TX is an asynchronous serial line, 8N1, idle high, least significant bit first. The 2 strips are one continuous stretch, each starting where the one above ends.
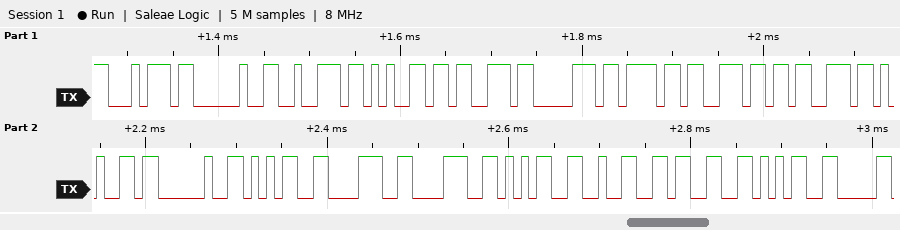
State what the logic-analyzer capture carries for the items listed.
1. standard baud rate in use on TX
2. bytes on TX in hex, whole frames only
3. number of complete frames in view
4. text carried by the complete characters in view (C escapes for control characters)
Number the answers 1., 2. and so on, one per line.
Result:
1. 115200 baud
2. 74 20 72 65 73 70 6F 6E 73 65 20 35 38 38 35 32 33 35
3. 18
4. "t response 5885235"
